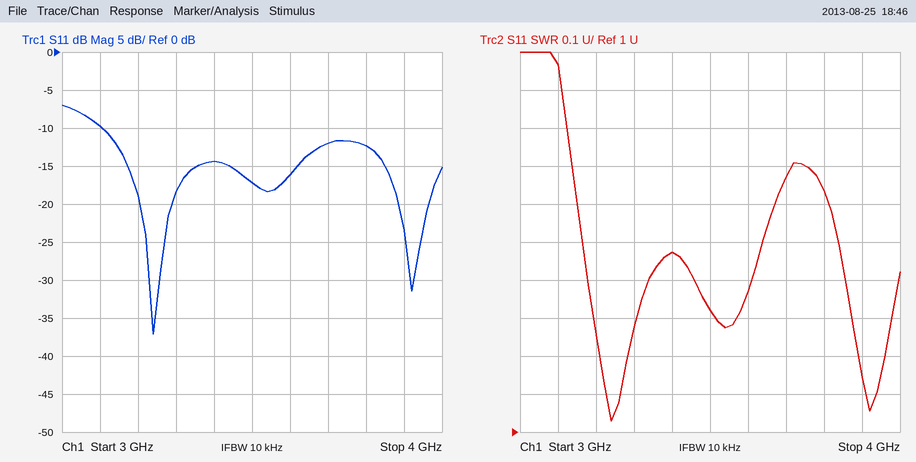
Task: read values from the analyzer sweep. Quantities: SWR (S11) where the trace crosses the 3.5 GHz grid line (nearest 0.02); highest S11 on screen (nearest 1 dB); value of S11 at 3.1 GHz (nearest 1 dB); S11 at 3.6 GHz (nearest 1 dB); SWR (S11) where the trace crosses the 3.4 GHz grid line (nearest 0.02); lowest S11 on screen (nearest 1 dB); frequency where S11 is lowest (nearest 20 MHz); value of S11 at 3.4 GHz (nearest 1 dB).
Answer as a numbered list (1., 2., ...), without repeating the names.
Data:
1. 1.32
2. -7 dB
3. -10 dB
4. -16 dB
5. 1.48
6. -37 dB
7. 3.24 GHz
8. -14 dB
